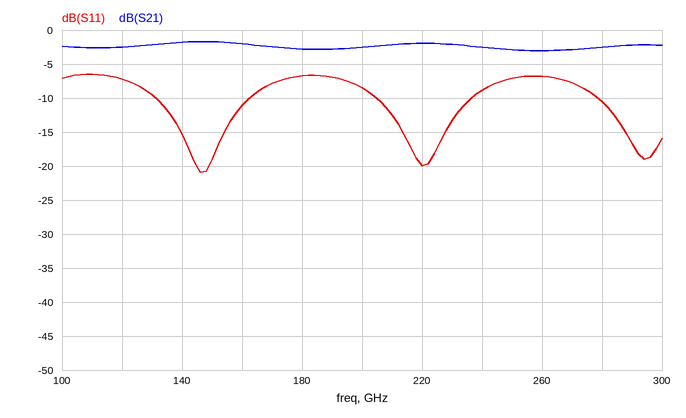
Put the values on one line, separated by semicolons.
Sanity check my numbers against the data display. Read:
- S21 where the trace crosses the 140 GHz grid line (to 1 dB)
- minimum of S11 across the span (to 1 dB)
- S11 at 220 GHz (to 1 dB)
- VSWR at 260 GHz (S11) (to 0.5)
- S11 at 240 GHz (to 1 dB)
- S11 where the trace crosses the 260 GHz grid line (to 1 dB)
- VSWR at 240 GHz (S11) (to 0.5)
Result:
-2 dB; -21 dB; -20 dB; 2.5; -9 dB; -7 dB; 2.0
